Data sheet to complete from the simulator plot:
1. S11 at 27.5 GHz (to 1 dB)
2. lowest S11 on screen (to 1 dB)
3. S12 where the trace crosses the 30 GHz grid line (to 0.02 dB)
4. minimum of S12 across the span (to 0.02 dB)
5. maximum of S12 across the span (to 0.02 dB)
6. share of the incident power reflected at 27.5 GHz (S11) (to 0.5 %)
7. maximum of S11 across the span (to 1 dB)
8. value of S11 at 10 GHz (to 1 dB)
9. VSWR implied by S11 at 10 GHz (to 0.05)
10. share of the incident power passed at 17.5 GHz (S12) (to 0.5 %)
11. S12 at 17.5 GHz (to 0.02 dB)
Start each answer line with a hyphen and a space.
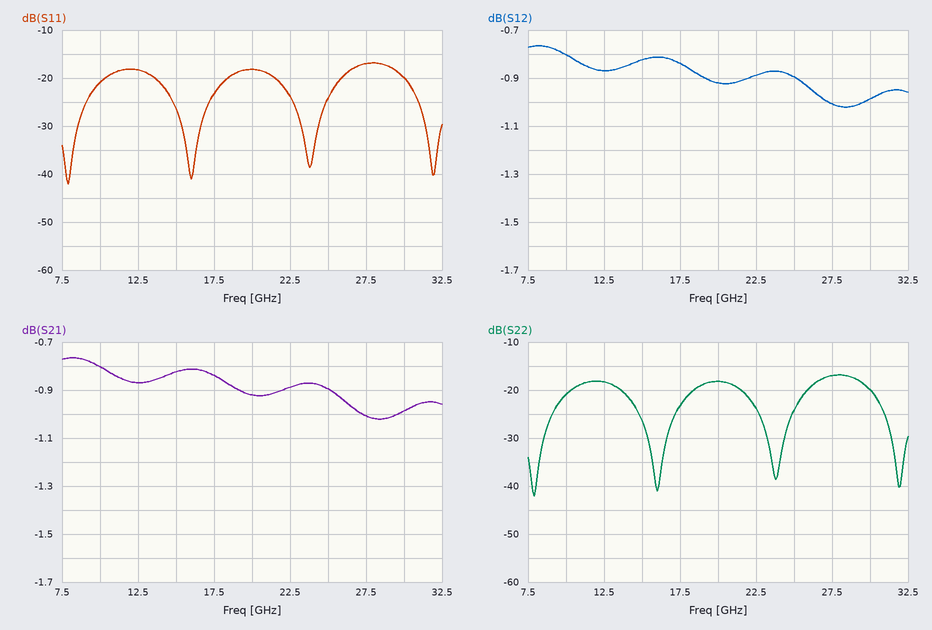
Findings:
- -17 dB
- -42 dB
- -0.98 dB
- -1.02 dB
- -0.76 dB
- 2.0 %
- -17 dB
- -21 dB
- 1.20
- 82.5 %
- -0.84 dB
